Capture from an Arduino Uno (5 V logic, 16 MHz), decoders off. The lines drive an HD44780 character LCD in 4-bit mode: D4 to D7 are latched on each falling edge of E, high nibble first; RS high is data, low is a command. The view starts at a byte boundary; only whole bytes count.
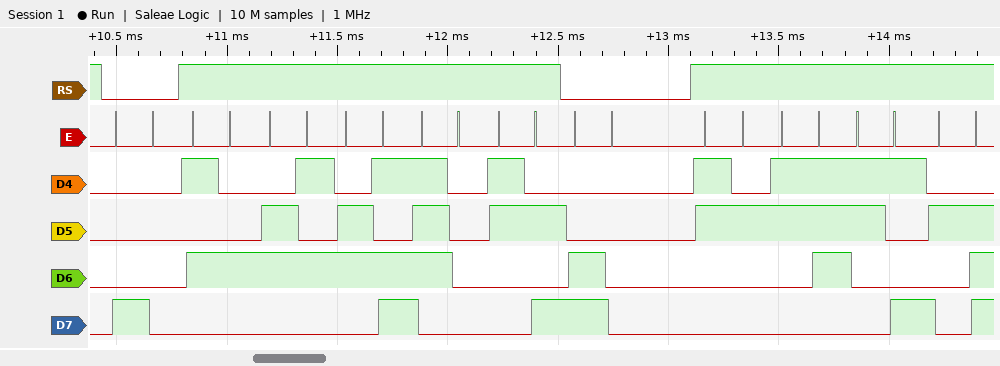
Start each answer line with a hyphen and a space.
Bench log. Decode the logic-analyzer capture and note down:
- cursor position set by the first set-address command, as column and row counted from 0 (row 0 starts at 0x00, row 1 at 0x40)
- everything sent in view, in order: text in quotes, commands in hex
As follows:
- column 0, row 0
- 0x80 "Temp:" 0xC0 "279."
